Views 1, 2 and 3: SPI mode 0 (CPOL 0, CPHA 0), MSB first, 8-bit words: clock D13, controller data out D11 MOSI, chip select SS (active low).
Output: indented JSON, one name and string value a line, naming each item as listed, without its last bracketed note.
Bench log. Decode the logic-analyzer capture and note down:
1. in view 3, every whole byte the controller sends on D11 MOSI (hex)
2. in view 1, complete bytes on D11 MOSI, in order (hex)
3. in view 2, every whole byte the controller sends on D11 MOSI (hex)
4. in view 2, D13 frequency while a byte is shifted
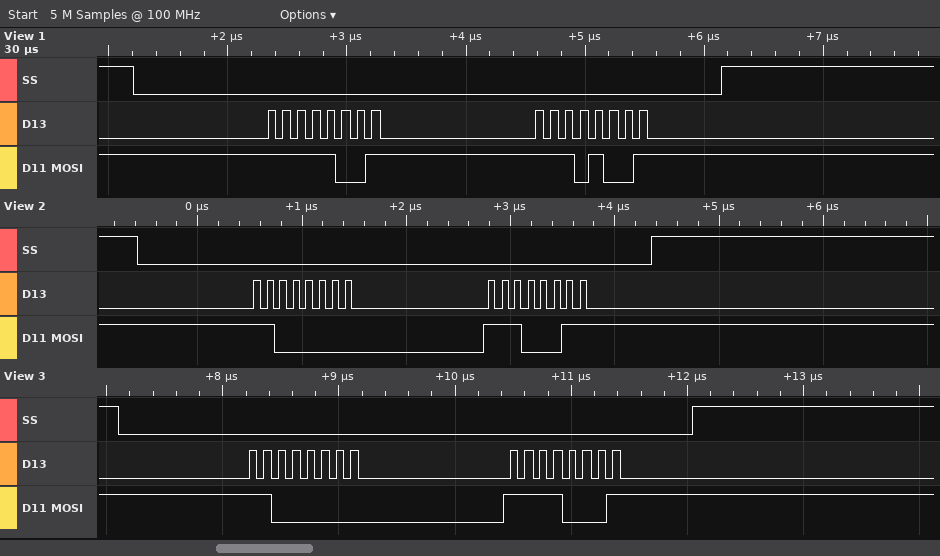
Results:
{
  "in view 3, every whole byte the controller sends on D11 MOSI": "0xC0 0xF1",
  "in view 1, complete bytes on D11 MOSI, in order": "F9 E9",
  "in view 2, every whole byte the controller sends on D11 MOSI": "C0 E3",
  "in view 2, D13 frequency while a byte is shifted": "8 MHz"
}
